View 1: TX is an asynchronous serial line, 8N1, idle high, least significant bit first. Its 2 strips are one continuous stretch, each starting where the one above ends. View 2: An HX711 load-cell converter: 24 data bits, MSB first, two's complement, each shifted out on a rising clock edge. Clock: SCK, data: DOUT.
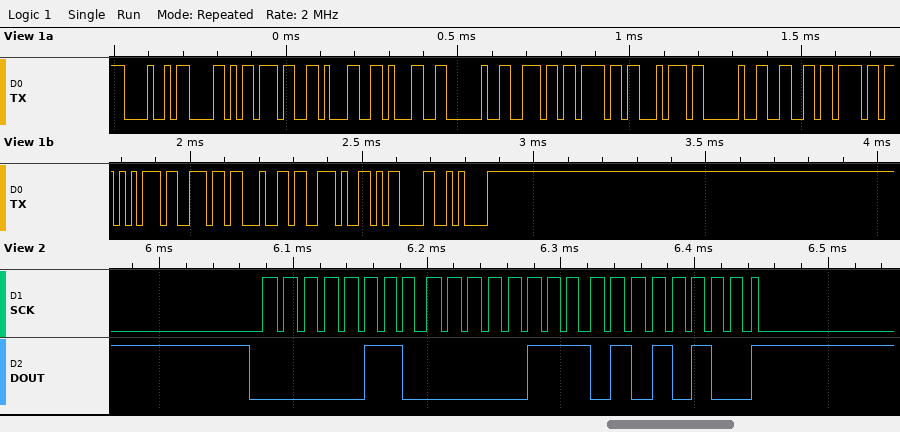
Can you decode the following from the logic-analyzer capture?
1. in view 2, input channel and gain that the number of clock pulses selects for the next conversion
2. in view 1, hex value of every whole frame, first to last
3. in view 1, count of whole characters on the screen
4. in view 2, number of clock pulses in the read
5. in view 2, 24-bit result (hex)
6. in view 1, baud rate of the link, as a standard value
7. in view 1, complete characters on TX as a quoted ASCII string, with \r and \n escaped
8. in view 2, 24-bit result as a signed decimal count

channel A, gain 128
48 58 37 31 31 20 6E 6F 74 20 66 6F 75 6E 64 2E 0D 0A
18
25
0x060754
57600 baud
"HX711 not found.\r\n"
395092
